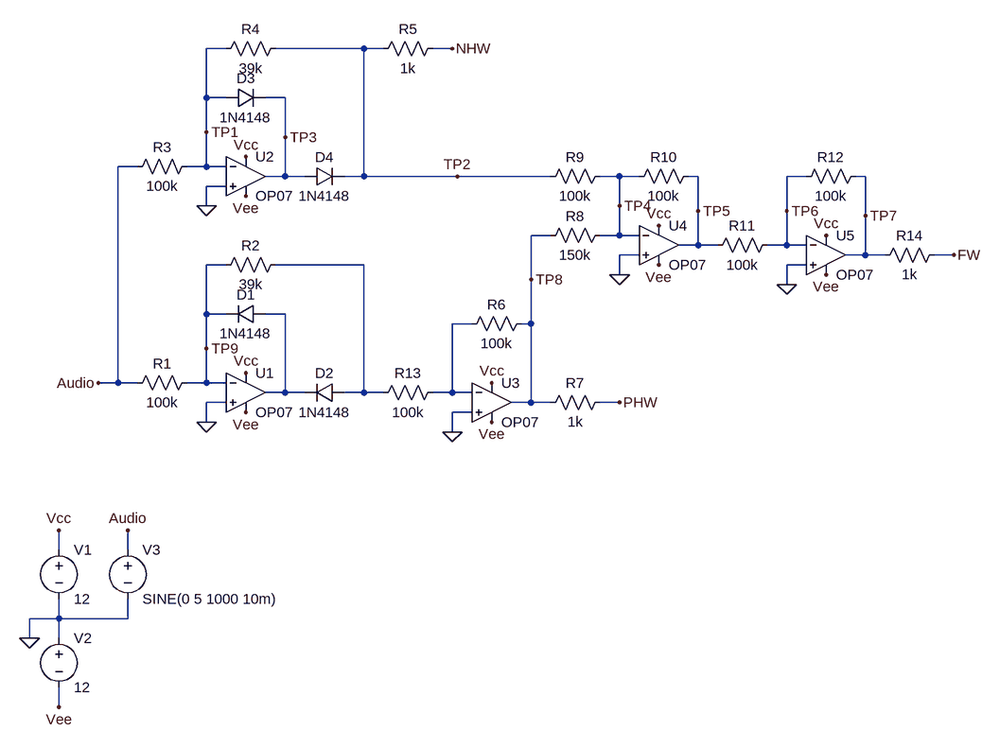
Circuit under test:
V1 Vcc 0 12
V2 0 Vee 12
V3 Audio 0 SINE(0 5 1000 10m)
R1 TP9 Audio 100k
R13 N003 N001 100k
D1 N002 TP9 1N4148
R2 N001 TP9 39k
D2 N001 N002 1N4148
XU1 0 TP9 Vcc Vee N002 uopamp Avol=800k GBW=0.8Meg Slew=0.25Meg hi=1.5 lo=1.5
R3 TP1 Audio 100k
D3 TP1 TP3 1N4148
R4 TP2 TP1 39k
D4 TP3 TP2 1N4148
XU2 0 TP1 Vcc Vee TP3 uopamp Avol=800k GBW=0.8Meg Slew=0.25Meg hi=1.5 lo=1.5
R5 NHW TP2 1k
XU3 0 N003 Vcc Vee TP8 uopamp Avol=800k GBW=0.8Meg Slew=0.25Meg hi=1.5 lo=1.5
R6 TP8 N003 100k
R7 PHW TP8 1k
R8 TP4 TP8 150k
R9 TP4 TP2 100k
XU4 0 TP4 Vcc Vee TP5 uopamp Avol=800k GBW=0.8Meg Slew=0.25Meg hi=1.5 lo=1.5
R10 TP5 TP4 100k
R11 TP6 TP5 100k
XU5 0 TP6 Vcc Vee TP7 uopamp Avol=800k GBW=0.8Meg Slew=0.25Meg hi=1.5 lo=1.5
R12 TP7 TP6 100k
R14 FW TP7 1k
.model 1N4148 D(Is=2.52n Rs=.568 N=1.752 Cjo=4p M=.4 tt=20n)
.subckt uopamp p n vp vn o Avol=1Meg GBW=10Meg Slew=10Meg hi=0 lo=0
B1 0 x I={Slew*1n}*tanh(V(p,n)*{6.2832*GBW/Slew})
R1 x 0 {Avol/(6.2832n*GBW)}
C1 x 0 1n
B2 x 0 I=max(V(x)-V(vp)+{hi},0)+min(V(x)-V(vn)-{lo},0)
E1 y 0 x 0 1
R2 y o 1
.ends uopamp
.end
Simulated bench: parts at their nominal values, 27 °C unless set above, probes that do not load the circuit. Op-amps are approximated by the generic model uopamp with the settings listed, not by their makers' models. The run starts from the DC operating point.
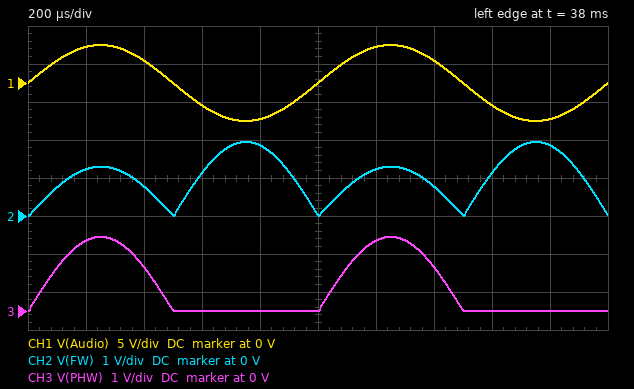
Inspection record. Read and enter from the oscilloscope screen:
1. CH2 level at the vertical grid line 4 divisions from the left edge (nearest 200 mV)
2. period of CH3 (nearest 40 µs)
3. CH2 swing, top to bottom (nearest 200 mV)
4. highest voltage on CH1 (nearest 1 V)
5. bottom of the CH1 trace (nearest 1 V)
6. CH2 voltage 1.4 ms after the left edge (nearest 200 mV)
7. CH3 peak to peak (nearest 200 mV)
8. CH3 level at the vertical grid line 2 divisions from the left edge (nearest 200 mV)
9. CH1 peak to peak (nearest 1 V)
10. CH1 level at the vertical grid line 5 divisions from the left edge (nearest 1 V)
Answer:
1.8 V
1.00 ms
2.0 V
5 V
-5 V
800 mV
2.0 V
1.2 V
10 V
0 V
